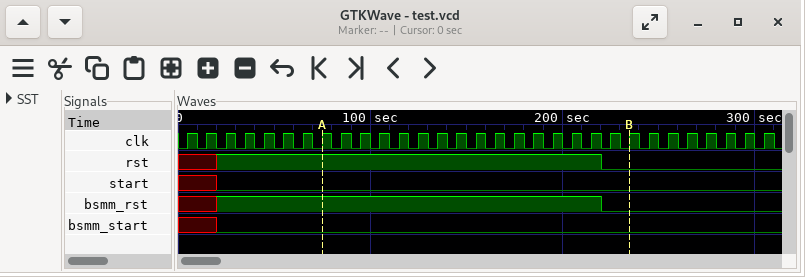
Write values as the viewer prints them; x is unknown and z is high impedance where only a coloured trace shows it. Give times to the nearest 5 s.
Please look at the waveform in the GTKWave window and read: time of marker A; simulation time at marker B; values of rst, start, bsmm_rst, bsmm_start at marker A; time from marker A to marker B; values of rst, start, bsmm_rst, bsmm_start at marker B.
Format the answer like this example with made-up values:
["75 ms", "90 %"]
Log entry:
["75 s", "235 s", "rst=1, start=0, bsmm_rst=1, bsmm_start=0", "160 s", "rst=0, start=0, bsmm_rst=0, bsmm_start=0"]
